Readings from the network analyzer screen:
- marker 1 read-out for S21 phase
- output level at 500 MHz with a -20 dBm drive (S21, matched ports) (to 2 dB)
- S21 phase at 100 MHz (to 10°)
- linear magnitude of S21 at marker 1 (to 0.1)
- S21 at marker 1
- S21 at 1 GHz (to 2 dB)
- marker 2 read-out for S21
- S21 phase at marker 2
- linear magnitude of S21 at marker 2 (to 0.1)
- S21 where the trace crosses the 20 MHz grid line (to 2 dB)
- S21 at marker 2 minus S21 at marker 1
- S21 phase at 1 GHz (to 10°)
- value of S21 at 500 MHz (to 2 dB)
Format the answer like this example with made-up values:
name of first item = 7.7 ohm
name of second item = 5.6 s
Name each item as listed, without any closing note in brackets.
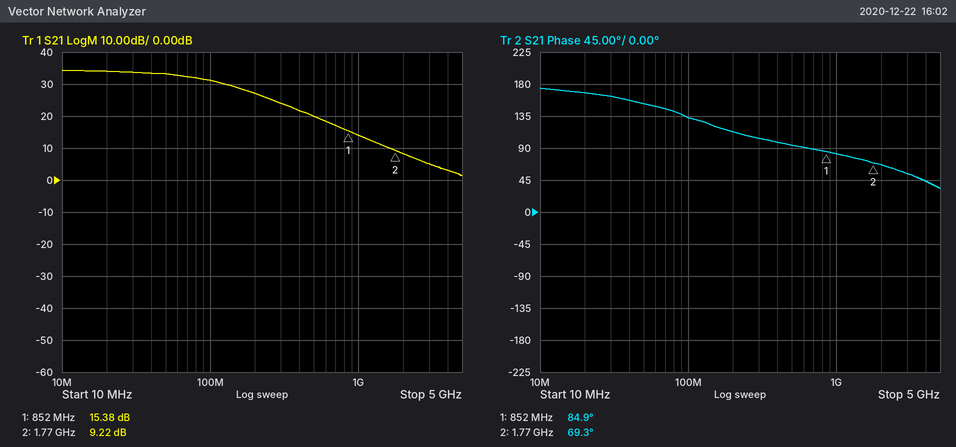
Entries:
marker 1 read-out for S21 phase = 84.9°
output level at 500 MHz with a -20 dBm drive (S21, matched ports) = 0 dBm
S21 phase at 100 MHz = 130°
linear magnitude of S21 at marker 1 = 5.9
S21 at marker 1 = 15.38 dB
S21 at 1 GHz = 14 dB
marker 2 read-out for S21 = 9.22 dB
S21 phase at marker 2 = 69.3°
linear magnitude of S21 at marker 2 = 2.9
S21 where the trace crosses the 20 MHz grid line = 34 dB
S21 at marker 2 minus S21 at marker 1 = -6.16 dB
S21 phase at 1 GHz = 80°
value of S21 at 500 MHz = 20 dB
